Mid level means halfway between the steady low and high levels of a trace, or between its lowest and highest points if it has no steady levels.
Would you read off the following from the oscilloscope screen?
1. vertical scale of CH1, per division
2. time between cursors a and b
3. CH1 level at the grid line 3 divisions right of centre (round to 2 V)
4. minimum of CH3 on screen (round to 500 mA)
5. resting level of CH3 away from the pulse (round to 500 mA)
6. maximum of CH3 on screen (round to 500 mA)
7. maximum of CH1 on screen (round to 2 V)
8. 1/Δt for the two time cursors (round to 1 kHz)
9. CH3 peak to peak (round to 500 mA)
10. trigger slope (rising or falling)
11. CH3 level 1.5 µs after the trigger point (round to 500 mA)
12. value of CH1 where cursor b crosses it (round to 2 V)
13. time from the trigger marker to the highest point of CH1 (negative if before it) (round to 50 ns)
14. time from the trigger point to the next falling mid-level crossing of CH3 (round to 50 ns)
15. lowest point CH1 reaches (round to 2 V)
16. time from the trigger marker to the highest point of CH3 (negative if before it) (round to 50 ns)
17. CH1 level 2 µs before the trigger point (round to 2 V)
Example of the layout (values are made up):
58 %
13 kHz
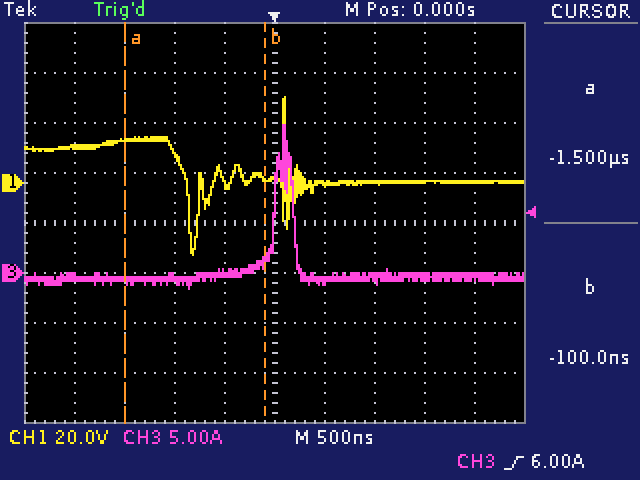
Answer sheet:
20 V
1.40 µs
0 V
-1.5 A
-500 mA
15.0 A
34 V
714 kHz
16.5 A
rising
-500 mA
2 V
+100 ns
200 ns
-28 V
+100 ns
14 V
